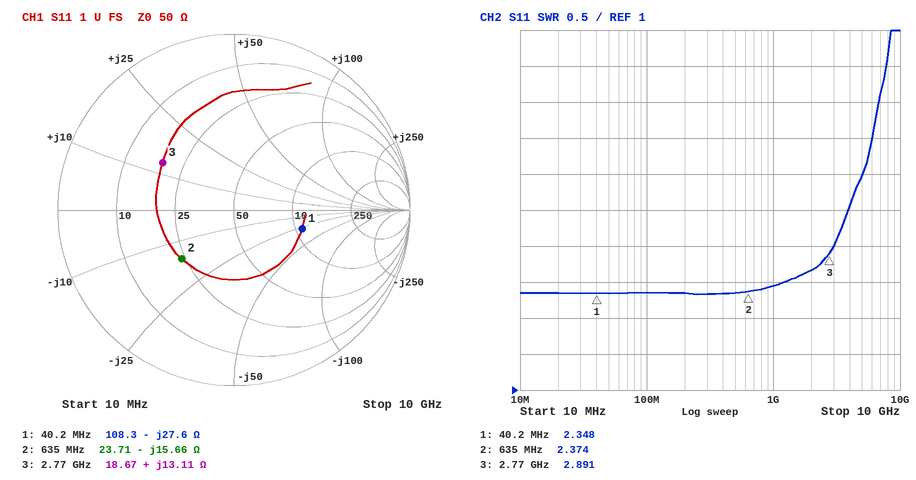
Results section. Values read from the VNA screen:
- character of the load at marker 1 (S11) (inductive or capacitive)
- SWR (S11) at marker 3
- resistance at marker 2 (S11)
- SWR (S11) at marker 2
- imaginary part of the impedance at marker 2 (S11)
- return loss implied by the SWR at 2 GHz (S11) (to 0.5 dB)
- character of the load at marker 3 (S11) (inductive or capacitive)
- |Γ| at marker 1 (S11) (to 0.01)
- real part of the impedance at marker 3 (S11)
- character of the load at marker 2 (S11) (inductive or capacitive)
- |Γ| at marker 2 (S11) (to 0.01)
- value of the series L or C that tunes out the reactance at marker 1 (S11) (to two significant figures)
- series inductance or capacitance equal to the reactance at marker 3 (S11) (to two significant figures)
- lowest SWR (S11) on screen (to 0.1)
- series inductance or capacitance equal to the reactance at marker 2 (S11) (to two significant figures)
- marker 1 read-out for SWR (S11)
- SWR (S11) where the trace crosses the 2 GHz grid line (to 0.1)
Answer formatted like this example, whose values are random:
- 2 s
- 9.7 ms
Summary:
- capacitive
- 2.891
- 23.71 Ω
- 2.374
- -15.66 Ω
- 7.0 dB
- inductive
- 0.40
- 18.67 Ω
- capacitive
- 0.41
- 110 nH
- 750 pH
- 2.3
- 16 pF
- 2.348
- 2.7
